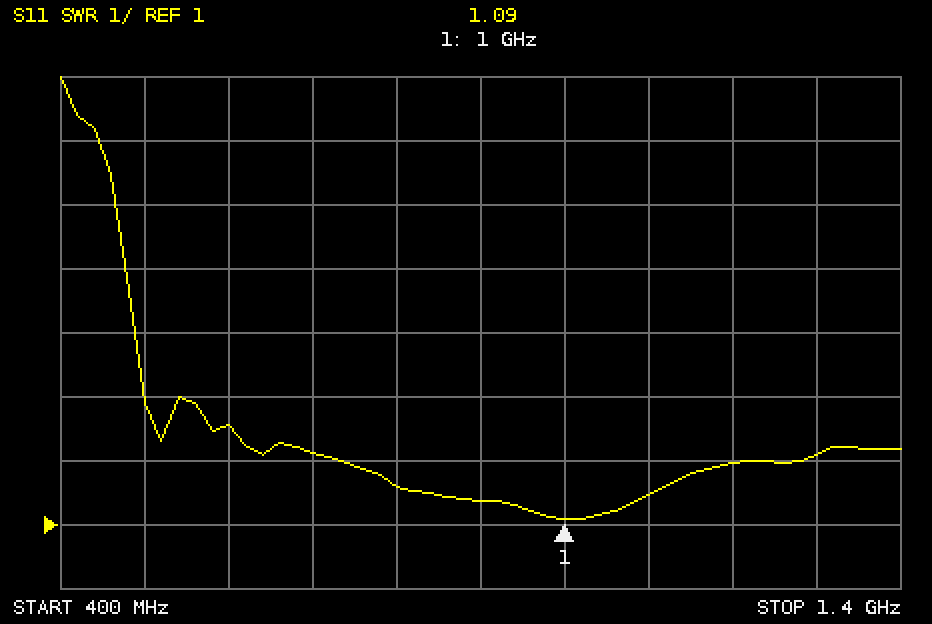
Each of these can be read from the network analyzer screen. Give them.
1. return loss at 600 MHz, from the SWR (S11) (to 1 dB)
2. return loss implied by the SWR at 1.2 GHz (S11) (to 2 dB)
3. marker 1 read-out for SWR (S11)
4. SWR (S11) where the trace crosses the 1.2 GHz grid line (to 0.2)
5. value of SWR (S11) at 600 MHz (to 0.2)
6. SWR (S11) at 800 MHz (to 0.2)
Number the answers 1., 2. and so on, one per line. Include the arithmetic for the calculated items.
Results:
1. −20 log10((2.6 − 1)/(2.6 + 1)) ≈ 7 dB
2. −20 log10((2 − 1)/(2 + 1)) ≈ 10 dB
3. 1.09
4. 2.0
5. 2.6
6. 1.6
